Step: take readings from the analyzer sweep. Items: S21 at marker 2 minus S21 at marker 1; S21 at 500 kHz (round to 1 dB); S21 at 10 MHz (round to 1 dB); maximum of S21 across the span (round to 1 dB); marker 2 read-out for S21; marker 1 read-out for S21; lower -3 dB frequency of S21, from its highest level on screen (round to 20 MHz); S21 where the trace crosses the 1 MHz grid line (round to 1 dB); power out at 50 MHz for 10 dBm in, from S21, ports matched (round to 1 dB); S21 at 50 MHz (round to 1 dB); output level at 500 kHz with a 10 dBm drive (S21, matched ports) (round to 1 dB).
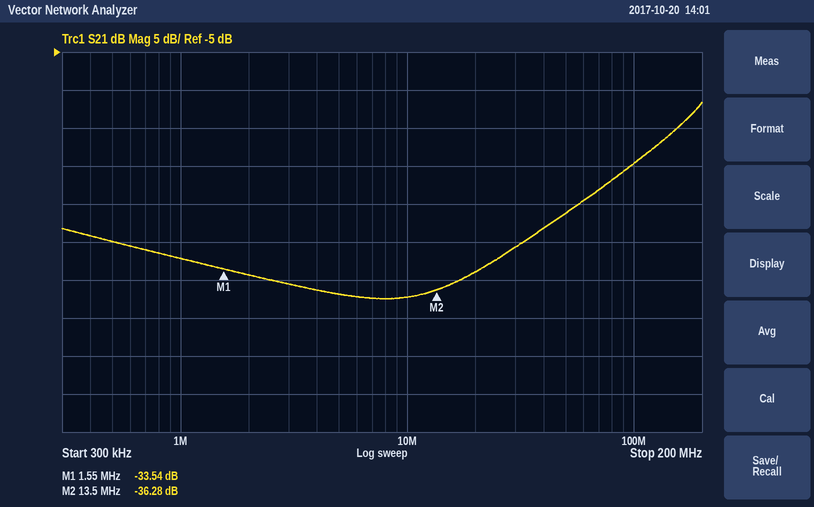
-2.74 dB
-30 dB
-37 dB
-12 dB
-36.28 dB
-33.54 dB
160 MHz
-32 dB
-16 dBm
-26 dB
-20 dBm
